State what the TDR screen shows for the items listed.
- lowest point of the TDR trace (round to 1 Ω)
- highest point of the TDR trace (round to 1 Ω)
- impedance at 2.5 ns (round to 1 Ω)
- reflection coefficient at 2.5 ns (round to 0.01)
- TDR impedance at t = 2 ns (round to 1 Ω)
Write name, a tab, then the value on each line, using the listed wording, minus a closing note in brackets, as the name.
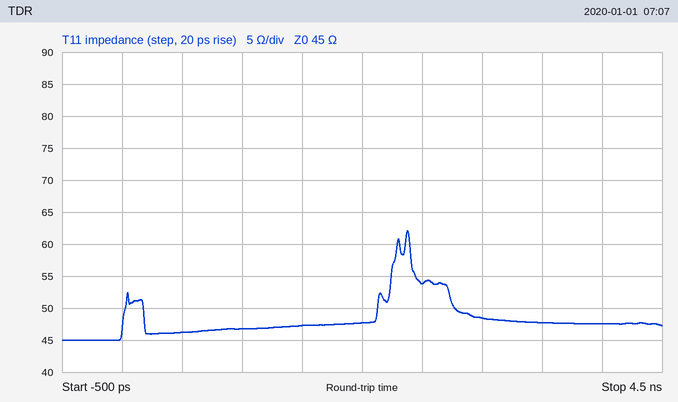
lowest point of the TDR trace	45 Ω
highest point of the TDR trace	62 Ω
impedance at 2.5 ns	54 Ω
reflection coefficient at 2.5 ns	+0.09
TDR impedance at t = 2 ns	48 Ω
